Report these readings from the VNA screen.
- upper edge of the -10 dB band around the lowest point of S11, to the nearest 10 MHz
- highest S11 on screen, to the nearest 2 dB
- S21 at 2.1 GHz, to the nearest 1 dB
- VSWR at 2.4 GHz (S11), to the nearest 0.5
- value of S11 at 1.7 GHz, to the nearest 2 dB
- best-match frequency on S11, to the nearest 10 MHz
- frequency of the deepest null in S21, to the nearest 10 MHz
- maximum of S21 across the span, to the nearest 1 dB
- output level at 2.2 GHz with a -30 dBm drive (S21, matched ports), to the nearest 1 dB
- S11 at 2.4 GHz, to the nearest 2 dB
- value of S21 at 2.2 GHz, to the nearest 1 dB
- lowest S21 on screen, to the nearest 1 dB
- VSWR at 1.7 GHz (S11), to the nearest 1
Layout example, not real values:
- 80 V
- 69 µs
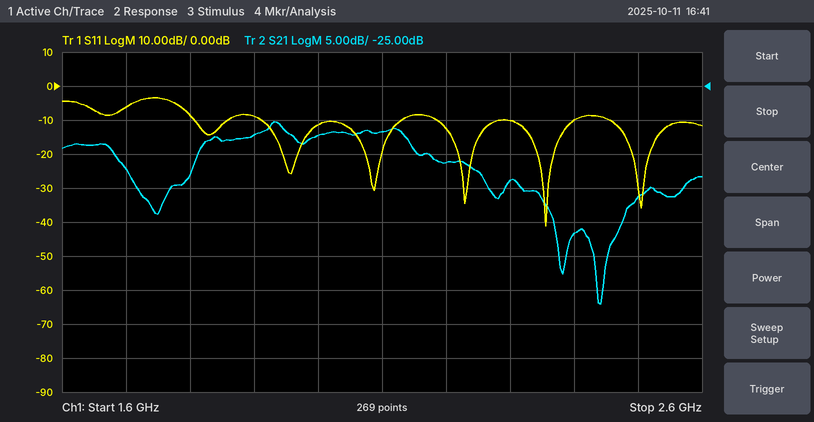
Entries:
- 2.40 GHz
- -4 dB
- -32 dB
- 2.0
- -6 dB
- 2.36 GHz
- 2.44 GHz
- -30 dB
- -66 dBm
- -10 dB
- -36 dB
- -57 dB
- 3
